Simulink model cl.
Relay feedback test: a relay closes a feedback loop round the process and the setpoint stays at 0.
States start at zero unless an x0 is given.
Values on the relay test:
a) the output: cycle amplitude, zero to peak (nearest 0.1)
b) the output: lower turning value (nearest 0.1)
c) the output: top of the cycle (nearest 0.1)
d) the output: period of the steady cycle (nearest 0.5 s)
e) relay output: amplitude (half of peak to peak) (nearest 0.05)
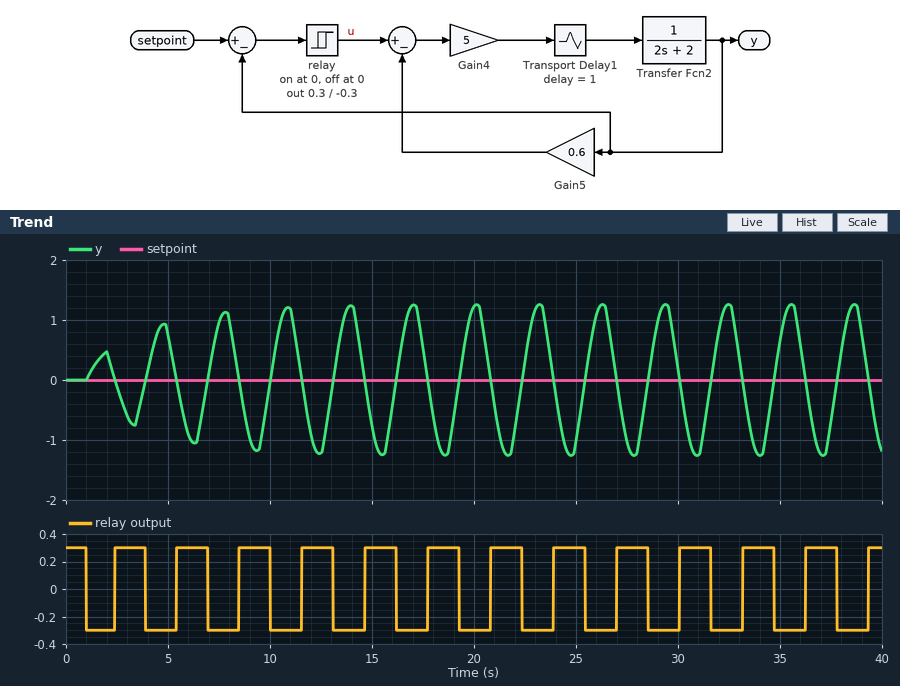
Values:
1.3
-1.3
1.3
3.0 s
0.30
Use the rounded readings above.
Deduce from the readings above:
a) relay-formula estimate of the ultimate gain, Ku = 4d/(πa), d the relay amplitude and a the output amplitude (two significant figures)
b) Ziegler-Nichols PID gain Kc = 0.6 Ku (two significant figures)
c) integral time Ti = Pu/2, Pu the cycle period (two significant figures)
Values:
0.29
0.17
1.5 s
